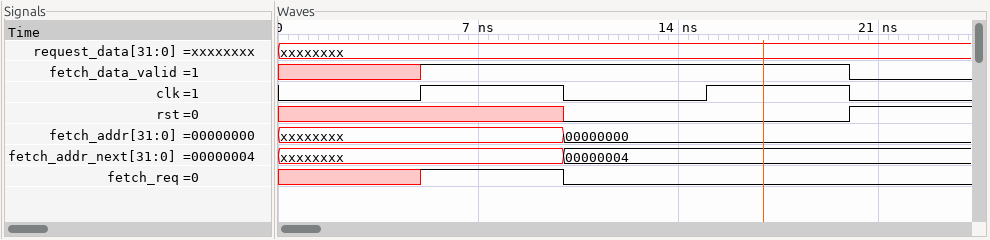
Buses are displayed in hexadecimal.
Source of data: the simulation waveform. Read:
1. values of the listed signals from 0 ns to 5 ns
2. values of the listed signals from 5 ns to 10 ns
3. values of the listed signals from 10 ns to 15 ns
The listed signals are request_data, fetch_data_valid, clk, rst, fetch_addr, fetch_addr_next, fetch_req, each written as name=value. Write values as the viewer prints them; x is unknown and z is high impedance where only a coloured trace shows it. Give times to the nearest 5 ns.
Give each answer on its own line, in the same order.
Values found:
request_data=xxxxxxxx, fetch_data_valid=x, clk=0, rst=x, fetch_addr=xxxxxxxx, fetch_addr_next=xxxxxxxx, fetch_req=x
request_data=xxxxxxxx, fetch_data_valid=1, clk=1, rst=x, fetch_addr=xxxxxxxx, fetch_addr_next=xxxxxxxx, fetch_req=1
request_data=xxxxxxxx, fetch_data_valid=1, clk=0, rst=0, fetch_addr=00000000, fetch_addr_next=00000004, fetch_req=0
